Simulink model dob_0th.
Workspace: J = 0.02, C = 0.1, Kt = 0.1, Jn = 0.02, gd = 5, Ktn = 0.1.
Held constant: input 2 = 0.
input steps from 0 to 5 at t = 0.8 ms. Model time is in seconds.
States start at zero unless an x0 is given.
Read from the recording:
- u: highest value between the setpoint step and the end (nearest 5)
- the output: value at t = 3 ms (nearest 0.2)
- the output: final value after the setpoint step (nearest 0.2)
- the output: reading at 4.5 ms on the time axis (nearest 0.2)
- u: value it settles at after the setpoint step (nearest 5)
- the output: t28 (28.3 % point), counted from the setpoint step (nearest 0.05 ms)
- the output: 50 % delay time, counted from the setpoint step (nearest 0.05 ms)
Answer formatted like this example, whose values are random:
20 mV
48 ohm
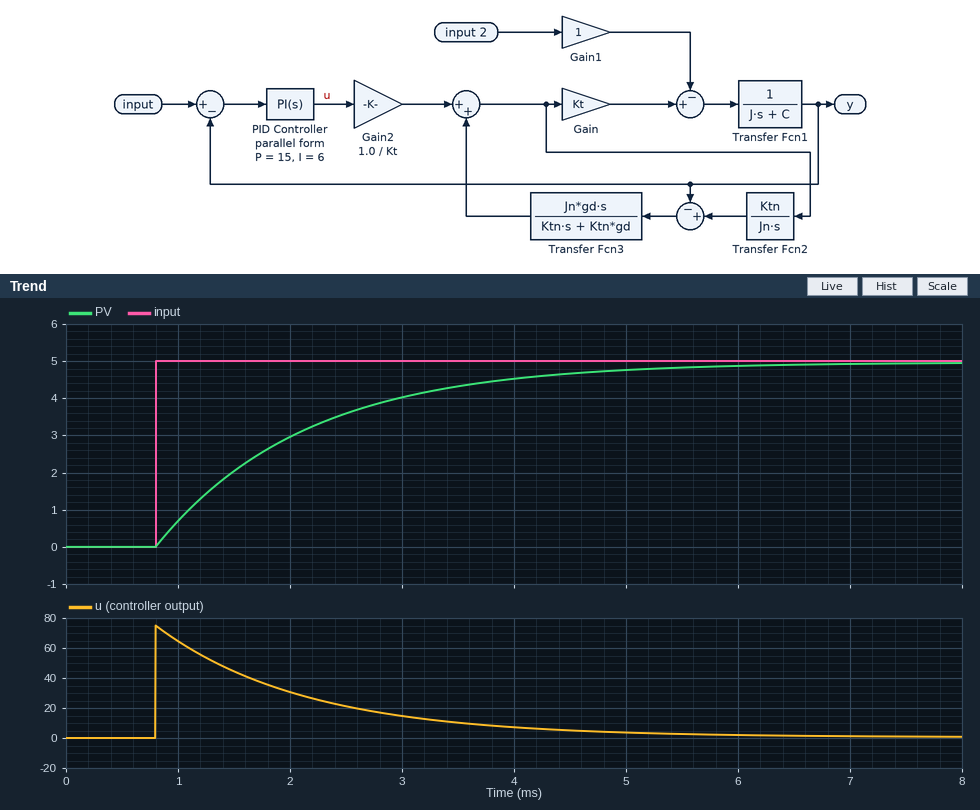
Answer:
75
4.0
5.0
4.6
0
0.45 ms
0.90 ms
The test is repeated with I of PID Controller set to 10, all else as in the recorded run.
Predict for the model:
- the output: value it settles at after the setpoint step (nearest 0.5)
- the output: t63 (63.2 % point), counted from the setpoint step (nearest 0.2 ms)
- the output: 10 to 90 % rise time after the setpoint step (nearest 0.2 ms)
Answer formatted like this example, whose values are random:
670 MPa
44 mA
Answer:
5.0
1.4 ms
3.0 ms
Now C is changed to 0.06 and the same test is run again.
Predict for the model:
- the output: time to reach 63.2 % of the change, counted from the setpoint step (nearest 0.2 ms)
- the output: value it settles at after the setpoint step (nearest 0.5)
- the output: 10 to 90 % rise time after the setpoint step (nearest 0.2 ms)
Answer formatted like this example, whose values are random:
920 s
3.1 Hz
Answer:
1.4 ms
5.0
3.0 ms
